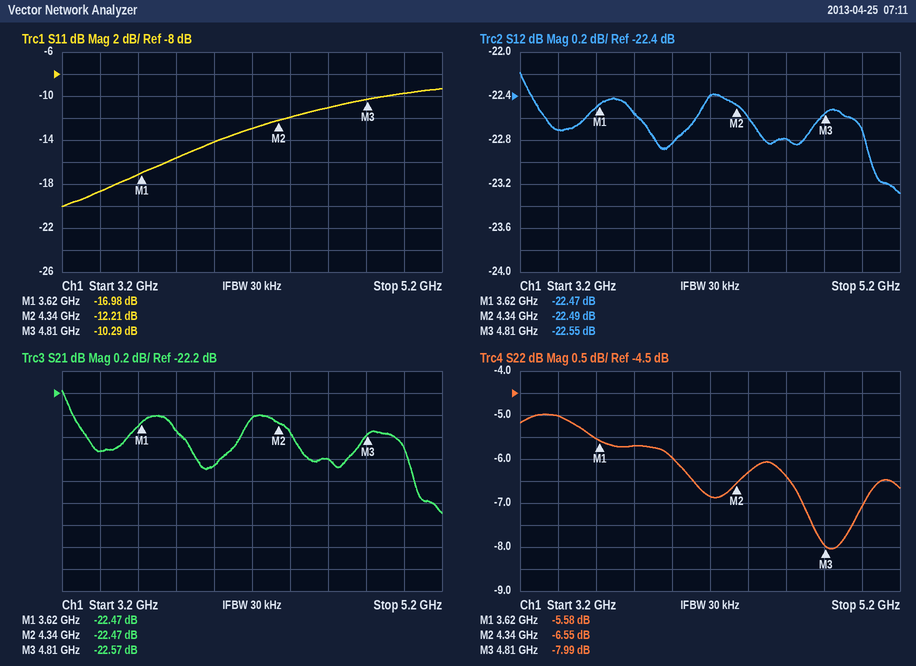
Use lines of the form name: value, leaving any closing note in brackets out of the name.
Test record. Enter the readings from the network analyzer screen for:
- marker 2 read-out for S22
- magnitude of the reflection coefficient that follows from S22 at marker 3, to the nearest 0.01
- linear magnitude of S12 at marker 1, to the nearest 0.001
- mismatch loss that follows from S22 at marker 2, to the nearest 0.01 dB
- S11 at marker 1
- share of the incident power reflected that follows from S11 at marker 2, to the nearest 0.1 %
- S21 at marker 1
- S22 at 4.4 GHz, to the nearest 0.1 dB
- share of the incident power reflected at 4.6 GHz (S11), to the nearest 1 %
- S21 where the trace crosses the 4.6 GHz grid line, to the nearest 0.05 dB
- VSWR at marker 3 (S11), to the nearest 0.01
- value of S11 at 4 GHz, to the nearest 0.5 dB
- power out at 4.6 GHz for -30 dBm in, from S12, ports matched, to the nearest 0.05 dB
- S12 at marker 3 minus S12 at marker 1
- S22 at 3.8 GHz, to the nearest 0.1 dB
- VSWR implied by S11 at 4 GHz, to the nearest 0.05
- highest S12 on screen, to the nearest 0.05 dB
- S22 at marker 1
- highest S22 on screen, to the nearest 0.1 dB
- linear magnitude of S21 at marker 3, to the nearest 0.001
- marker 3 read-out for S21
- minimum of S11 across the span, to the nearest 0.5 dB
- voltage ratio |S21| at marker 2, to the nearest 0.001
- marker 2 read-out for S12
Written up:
marker 2 read-out for S22: -6.55 dB
magnitude of the reflection coefficient that follows from S22 at marker 3, to the nearest 0.01: 0.40
linear magnitude of S12 at marker 1, to the nearest 0.001: 0.075
mismatch loss that follows from S22 at marker 2, to the nearest 0.01 dB: 1.09 dB
S11 at marker 1: -16.98 dB
share of the incident power reflected that follows from S11 at marker 2, to the nearest 0.1 %: 6.0 %
S21 at marker 1: -22.47 dB
S22 at 4.4 GHz, to the nearest 0.1 dB: -6.3 dB
share of the incident power reflected at 4.6 GHz (S11), to the nearest 1 %: 8 %
S21 where the trace crosses the 4.6 GHz grid line, to the nearest 0.05 dB: -22.80 dB
VSWR at marker 3 (S11), to the nearest 0.01: 1.88
value of S11 at 4 GHz, to the nearest 0.5 dB: -14.0 dB
power out at 4.6 GHz for -30 dBm in, from S12, ports matched, to the nearest 0.05 dB: -52.80 dBm
S12 at marker 3 minus S12 at marker 1: -0.08 dB
S22 at 3.8 GHz, to the nearest 0.1 dB: -5.7 dB
VSWR implied by S11 at 4 GHz, to the nearest 0.05: 1.50
highest S12 on screen, to the nearest 0.05 dB: -22.20 dB
S22 at marker 1: -5.58 dB
highest S22 on screen, to the nearest 0.1 dB: -5.0 dB
linear magnitude of S21 at marker 3, to the nearest 0.001: 0.074
marker 3 read-out for S21: -22.57 dB
minimum of S11 across the span, to the nearest 0.5 dB: -20.0 dB
voltage ratio |S21| at marker 2, to the nearest 0.001: 0.075
marker 2 read-out for S12: -22.49 dB
